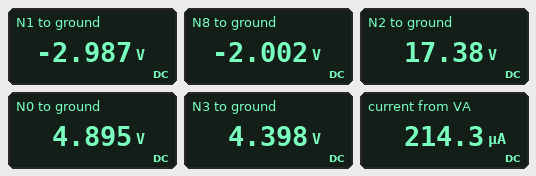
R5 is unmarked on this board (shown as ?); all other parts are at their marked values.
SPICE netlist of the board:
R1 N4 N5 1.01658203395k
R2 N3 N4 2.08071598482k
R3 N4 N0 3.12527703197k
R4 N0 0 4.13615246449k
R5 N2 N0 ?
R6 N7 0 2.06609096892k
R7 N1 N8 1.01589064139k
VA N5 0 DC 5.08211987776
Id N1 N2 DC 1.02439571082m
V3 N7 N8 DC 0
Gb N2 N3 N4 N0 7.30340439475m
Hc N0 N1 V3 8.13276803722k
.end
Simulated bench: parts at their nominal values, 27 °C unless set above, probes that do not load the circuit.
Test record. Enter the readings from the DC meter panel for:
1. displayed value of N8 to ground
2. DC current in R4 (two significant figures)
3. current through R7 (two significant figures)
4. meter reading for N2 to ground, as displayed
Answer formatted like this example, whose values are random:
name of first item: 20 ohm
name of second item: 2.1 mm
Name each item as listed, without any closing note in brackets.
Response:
displayed value of N8 to ground: -2.002 V
DC current in R4: 1.2 mA
current through R7: 970 µA
meter reading for N2 to ground, as displayed: 17.38 V
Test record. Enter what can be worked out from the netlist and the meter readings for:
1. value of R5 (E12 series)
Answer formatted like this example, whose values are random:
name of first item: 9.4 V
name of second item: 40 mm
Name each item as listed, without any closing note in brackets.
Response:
value of R5: 10 kΩ
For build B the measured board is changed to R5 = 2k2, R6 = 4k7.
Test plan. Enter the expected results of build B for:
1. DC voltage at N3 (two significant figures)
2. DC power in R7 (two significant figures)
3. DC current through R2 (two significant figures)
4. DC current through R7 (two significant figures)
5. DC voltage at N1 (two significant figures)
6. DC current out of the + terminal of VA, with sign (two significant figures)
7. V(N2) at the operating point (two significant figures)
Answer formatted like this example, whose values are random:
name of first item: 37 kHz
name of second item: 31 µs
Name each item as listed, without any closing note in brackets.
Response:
DC voltage at N3: 8.4 V
DC power in R7: 6.2 mW
DC current through R2: 1.1 mA
DC current through R7: 2.5 mA
DC voltage at N1: -14 V
DC current out of the + terminal of VA, with sign: -1.0 mA
V(N2) at the operating point: 5.9 V
